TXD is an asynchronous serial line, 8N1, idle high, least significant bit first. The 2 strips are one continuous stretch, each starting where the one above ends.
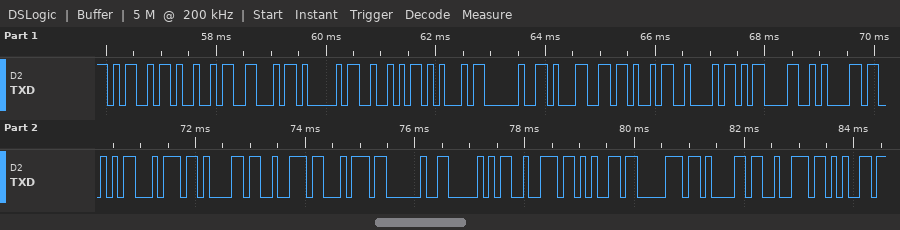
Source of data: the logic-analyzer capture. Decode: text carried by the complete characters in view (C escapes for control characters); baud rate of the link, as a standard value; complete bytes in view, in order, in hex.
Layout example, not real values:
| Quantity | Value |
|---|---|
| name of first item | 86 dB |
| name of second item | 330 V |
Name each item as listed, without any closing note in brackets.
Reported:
| Quantity | Value |
|---|---|
| text carried by the complete characters in view | "MIFARE 1KB\r\nStart Prepare" |
| baud rate of the link, as a standard value | 9600 baud |
| complete bytes in view, in order, in hex | 0x4D 0x49 0x46 0x41 0x52 0x45 0x20 0x31 0x4B 0x42 0x0D 0x0A 0x53 0x74 0x61 0x72 0x74 0x20 0x50 0x72 0x65 0x70 0x61 0x72 0x65 |
